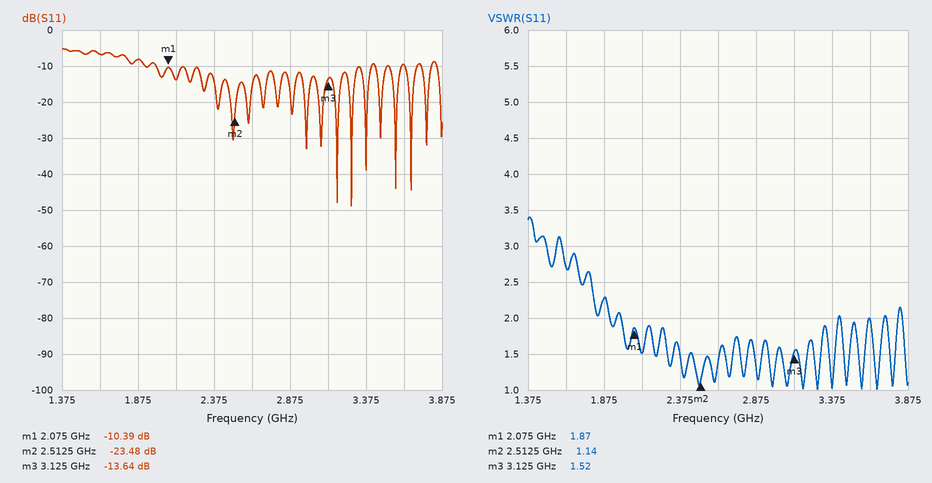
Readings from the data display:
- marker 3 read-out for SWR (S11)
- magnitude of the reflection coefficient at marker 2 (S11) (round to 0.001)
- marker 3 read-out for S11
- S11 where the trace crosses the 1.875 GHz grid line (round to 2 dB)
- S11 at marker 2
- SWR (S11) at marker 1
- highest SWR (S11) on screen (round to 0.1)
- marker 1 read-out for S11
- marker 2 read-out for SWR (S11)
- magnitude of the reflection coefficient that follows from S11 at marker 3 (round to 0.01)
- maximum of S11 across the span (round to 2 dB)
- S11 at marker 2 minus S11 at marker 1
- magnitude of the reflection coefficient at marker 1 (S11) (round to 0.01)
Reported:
1.52
0.067
-13.64 dB
-8 dB
-23.48 dB
1.87
3.4
-10.39 dB
1.14
0.21
-6 dB
-13.09 dB
0.30
